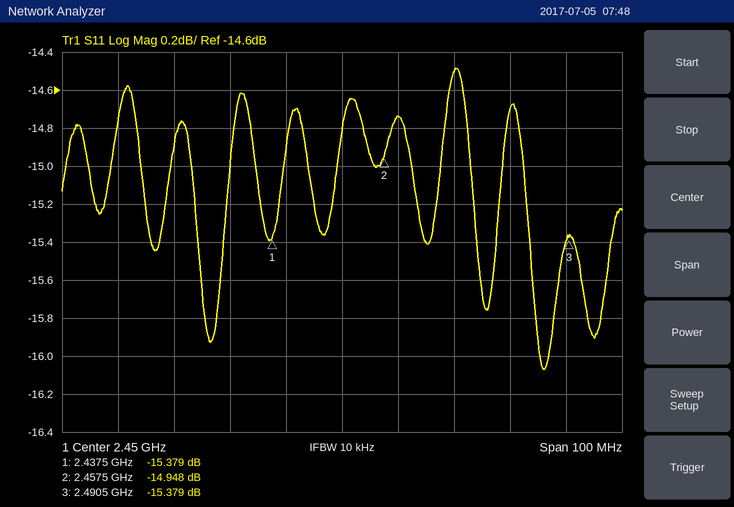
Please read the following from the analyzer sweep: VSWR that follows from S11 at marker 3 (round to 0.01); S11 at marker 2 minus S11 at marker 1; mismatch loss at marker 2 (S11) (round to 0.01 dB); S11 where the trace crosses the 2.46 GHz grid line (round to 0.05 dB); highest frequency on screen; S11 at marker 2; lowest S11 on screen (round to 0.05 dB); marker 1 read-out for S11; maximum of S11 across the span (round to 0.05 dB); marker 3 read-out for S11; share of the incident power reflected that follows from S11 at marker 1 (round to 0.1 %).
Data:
1.41
0.431 dB
0.14 dB
-14.75 dB
2.5 GHz
-14.948 dB
-16.05 dB
-15.379 dB
-14.50 dB
-15.379 dB
2.9 %
